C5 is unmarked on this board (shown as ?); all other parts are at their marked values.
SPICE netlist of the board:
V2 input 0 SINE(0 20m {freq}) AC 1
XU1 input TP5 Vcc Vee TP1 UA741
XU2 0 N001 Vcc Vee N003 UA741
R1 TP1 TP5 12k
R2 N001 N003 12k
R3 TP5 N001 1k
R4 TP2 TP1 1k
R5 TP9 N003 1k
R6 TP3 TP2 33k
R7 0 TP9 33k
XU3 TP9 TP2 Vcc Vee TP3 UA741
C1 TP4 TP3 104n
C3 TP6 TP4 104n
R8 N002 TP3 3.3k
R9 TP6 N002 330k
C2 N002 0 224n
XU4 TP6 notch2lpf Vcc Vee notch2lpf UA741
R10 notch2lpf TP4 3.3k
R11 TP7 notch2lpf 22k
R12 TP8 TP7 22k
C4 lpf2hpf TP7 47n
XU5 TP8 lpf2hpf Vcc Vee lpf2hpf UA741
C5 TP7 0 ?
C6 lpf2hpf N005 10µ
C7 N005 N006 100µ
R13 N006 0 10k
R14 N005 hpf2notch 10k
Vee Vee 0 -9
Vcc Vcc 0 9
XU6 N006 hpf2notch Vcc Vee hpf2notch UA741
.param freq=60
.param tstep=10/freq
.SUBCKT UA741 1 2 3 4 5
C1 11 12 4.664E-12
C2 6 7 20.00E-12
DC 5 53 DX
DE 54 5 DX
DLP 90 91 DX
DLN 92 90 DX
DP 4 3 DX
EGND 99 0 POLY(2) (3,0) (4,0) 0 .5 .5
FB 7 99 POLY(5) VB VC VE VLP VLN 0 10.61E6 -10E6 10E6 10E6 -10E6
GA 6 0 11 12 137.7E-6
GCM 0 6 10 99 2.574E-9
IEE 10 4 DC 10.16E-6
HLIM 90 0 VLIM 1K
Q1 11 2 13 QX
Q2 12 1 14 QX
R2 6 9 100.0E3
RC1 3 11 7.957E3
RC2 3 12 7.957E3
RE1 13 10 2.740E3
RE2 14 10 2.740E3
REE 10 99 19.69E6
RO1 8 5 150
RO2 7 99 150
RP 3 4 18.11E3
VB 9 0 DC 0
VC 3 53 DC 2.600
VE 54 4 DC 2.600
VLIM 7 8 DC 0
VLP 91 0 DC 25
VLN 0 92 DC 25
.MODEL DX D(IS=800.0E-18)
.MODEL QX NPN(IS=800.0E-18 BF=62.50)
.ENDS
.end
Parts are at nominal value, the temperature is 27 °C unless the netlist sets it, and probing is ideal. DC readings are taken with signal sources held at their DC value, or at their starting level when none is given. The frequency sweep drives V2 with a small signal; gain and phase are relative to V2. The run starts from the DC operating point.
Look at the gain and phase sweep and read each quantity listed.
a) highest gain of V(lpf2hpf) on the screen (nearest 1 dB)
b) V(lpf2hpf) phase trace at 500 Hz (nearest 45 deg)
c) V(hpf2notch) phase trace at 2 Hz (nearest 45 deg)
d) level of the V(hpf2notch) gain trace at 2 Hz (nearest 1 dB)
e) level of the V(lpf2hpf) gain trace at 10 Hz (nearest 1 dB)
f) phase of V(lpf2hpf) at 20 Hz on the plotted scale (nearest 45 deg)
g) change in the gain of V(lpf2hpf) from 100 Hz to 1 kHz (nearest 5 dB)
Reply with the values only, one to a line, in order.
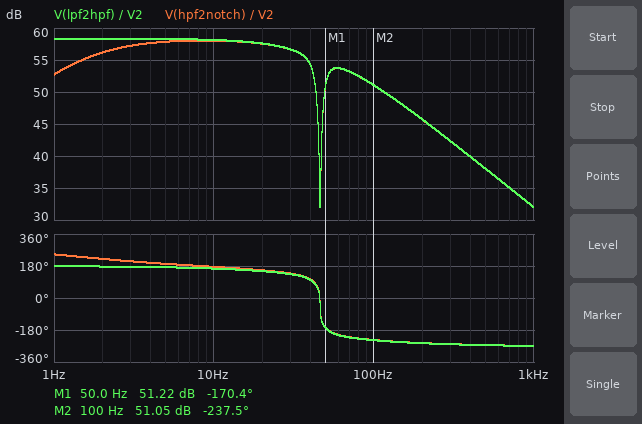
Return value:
58 dB
-270 deg
225 deg
56 dB
58 dB
135 deg
-20 dB
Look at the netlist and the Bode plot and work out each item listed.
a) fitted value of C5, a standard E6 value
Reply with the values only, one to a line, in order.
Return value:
150 nF
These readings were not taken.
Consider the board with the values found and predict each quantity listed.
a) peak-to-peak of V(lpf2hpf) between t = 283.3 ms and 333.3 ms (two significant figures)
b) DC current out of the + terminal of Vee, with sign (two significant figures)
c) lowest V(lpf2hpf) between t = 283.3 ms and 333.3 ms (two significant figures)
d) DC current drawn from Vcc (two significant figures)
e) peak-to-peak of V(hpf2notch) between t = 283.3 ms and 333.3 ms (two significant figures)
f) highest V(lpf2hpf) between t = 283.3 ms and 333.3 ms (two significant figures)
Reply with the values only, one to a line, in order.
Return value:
6.7 V
-6.0 mA
-3.4 V
6.0 mA
6.7 V
3.3 V
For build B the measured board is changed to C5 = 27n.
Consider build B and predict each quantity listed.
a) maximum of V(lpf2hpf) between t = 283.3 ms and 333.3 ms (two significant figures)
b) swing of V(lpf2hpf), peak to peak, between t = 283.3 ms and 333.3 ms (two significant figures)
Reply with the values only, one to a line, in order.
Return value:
6.5 V
13 V
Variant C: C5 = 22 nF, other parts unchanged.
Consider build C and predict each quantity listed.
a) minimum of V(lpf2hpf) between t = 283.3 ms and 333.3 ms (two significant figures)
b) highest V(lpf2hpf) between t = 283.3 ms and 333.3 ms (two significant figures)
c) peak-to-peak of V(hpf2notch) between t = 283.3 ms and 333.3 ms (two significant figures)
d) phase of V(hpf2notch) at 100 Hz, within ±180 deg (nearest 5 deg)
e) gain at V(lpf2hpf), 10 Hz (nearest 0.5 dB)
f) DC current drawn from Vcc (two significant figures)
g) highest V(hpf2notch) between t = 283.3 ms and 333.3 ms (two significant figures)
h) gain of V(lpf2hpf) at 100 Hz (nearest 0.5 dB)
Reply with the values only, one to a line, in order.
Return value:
-6.7 V
6.7 V
14 V
170 deg
58.5 dB
6.0 mA
6.8 V
58.0 dB
